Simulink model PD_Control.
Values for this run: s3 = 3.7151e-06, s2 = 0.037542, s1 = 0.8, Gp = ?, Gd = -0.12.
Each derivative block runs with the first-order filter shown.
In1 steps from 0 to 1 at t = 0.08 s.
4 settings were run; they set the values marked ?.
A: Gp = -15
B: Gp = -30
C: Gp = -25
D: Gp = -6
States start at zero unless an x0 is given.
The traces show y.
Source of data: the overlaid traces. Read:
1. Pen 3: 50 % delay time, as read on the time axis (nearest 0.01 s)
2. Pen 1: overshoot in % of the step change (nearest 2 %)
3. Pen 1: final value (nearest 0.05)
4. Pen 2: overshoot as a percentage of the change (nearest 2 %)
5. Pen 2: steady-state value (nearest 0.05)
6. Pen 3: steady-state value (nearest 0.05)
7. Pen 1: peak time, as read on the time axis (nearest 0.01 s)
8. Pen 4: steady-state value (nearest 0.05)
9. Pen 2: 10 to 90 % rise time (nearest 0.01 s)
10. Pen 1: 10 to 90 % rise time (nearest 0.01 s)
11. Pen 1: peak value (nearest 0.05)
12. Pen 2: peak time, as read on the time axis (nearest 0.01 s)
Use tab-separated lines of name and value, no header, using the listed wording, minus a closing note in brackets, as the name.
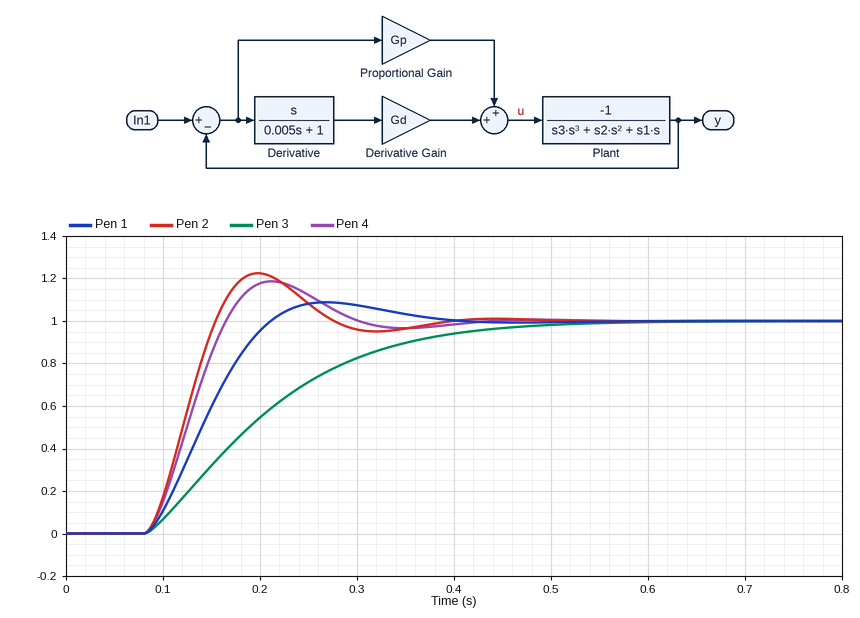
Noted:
Pen 3: 50 % delay time, as read on the time axis	0.19 s
Pen 1: overshoot in % of the step change	8 %
Pen 1: final value	1.00
Pen 2: overshoot as a percentage of the change	22 %
Pen 2: steady-state value	1.00
Pen 3: steady-state value	1.00
Pen 1: peak time, as read on the time axis	0.27 s
Pen 4: steady-state value	1.00
Pen 2: 10 to 90 % rise time	0.05 s
Pen 1: 10 to 90 % rise time	0.09 s
Pen 1: peak value	1.10
Pen 2: peak time, as read on the time axis	0.20 s
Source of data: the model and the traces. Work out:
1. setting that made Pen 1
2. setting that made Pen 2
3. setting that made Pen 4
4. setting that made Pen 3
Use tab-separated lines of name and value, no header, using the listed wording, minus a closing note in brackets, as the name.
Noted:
setting that made Pen 1	A
setting that made Pen 2	B
setting that made Pen 4	C
setting that made Pen 3	D
